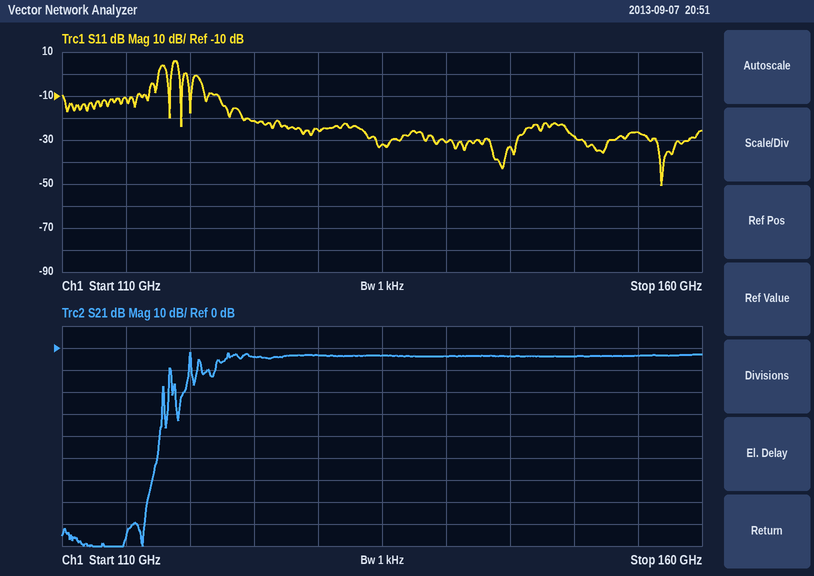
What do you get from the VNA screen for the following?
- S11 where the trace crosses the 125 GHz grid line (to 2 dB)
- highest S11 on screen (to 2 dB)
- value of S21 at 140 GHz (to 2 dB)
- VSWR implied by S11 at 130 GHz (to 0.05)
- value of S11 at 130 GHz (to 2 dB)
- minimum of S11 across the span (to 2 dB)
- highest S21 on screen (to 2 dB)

-22 dB
6 dB
-4 dB
1.10
-26 dB
-50 dB
-2 dB
